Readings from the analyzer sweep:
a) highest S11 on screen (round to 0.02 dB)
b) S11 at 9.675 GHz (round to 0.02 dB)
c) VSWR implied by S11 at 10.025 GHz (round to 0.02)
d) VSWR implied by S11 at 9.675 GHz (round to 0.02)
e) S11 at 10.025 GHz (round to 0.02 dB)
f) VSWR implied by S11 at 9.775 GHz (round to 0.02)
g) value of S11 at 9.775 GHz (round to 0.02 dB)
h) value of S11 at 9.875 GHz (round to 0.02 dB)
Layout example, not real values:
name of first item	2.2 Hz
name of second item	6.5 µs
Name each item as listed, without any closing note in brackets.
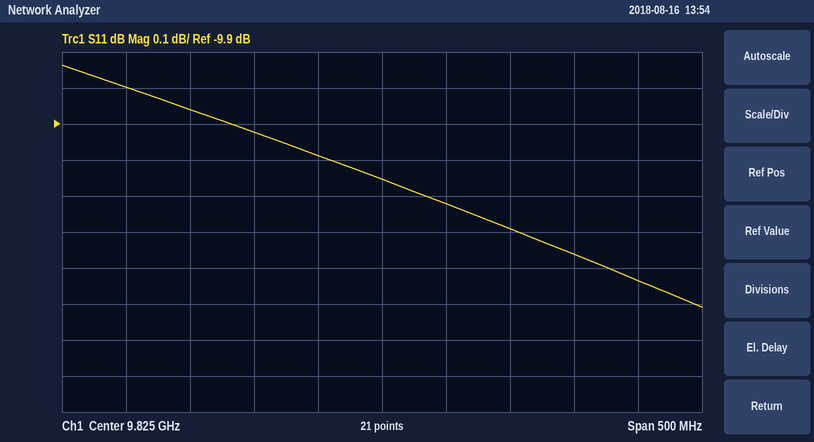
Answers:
highest S11 on screen	-9.74 dB
S11 at 9.675 GHz	-9.86 dB
VSWR implied by S11 at 10.025 GHz	1.88
VSWR implied by S11 at 9.675 GHz	1.94
S11 at 10.025 GHz	-10.34 dB
VSWR implied by S11 at 9.775 GHz	1.92
value of S11 at 9.775 GHz	-9.98 dB
value of S11 at 9.875 GHz	-10.12 dB
